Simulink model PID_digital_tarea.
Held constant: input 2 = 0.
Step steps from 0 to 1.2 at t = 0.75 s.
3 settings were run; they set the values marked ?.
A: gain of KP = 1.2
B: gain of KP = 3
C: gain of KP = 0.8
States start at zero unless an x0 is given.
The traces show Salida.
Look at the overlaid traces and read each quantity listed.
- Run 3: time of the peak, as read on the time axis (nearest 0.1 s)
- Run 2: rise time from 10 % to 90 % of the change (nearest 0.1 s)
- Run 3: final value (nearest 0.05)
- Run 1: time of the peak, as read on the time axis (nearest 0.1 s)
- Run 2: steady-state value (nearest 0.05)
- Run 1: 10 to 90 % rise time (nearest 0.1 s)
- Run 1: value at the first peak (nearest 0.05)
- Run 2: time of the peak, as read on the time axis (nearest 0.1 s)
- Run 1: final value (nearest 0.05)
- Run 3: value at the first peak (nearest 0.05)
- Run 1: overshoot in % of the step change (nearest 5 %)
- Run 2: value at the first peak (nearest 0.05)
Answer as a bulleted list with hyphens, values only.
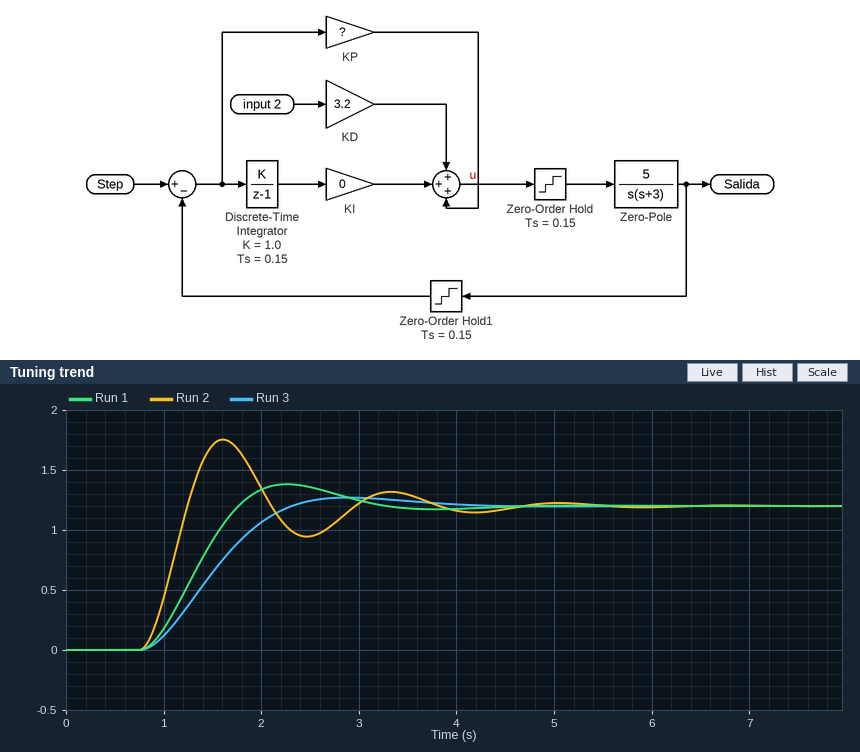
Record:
- 2.9 s
- 0.3 s
- 1.20
- 2.3 s
- 1.20
- 0.7 s
- 1.40
- 1.6 s
- 1.20
- 1.25
- 15 %
- 1.75
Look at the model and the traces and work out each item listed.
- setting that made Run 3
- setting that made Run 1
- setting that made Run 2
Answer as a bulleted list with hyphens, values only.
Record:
- C
- A
- B
